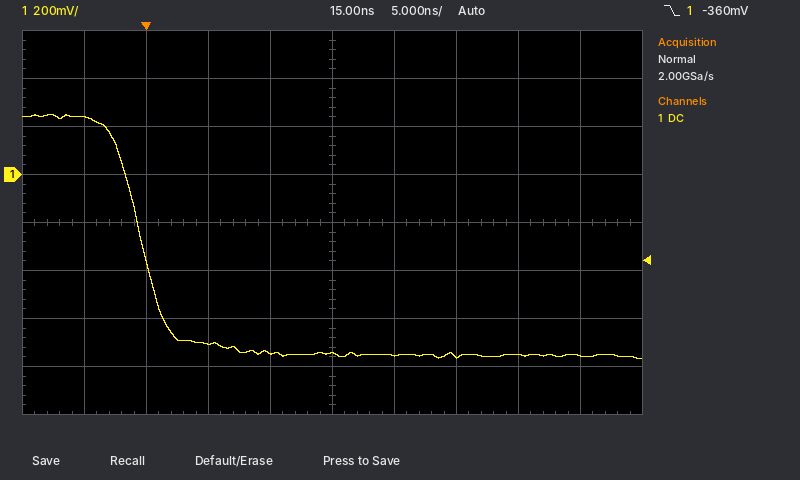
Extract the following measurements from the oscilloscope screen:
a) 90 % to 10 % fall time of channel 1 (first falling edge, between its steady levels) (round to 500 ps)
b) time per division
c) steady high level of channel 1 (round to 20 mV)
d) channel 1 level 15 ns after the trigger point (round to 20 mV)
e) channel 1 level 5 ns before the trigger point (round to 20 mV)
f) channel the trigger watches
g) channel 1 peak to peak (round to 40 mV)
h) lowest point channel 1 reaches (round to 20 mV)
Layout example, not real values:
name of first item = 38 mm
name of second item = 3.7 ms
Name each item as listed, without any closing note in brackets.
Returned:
90 % to 10 % fall time of channel 1 (first falling edge, between its steady levels) = 4.5 ns
time per division = 5 ns
steady high level of channel 1 = 240 mV
channel 1 level 15 ns after the trigger point = -740 mV
channel 1 level 5 ns before the trigger point = 240 mV
channel the trigger watches = channel 1
channel 1 peak to peak = 1.00 V
lowest point channel 1 reaches = -760 mV
